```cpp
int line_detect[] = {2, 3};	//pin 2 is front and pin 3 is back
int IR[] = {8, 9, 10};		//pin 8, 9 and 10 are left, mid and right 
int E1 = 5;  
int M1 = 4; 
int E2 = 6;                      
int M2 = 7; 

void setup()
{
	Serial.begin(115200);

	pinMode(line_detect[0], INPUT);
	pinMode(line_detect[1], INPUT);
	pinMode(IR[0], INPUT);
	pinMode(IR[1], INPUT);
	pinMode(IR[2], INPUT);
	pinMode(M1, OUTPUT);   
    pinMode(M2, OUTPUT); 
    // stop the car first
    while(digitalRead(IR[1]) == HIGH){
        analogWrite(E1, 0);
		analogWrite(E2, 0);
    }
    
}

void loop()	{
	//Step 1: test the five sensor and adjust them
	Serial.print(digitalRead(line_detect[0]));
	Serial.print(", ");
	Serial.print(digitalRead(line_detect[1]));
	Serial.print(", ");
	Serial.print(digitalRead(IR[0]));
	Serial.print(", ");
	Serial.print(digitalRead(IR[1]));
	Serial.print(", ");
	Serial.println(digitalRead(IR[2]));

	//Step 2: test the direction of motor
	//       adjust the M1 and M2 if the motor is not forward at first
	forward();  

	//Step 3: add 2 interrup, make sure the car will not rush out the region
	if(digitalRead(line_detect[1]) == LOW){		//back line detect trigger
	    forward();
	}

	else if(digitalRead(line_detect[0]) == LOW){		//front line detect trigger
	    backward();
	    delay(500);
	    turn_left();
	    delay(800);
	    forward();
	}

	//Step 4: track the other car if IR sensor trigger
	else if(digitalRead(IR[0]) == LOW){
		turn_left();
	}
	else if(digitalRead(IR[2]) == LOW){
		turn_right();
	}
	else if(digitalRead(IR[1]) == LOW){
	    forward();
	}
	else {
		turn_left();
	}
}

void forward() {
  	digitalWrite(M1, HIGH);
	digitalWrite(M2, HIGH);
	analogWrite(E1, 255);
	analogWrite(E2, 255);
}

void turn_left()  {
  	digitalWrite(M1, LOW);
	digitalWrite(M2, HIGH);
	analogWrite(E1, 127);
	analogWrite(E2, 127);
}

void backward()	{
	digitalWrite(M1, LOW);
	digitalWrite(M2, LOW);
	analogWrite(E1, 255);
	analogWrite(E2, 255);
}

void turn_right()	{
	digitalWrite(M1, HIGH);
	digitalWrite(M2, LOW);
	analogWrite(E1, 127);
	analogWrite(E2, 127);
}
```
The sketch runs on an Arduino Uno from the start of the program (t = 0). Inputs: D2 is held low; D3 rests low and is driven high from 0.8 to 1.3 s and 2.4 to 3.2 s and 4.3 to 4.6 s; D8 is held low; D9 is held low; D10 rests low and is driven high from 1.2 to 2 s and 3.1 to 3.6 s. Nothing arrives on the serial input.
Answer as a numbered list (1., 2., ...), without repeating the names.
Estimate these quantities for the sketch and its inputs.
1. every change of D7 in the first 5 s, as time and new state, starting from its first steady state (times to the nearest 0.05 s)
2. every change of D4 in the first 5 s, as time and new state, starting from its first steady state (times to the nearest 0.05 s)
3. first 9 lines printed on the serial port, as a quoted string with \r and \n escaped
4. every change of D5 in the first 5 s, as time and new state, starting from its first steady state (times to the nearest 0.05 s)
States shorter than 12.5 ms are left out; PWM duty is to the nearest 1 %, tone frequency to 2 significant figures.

1. 0 s high; 0.8 s low; 1.3 s high; 2.4 s low; 2.9 s high; 4.3 s low; 4.8 s high
2. 0 s high; 0.8 s low; 2.1 s high; 2.4 s low; 3.7 s high; 4.3 s low
3. "0, 0, 0, 0, 0\r\n0, 0, 0, 0, 0\r\n0, 0, 0, 0, 0\r\n0, 0, 0, 0, 0\r\n0, 0, 0, 0, 0\r\n0, 0, 0, 0, 0\r\n0, 0, 0, 0, 0\r\n0, 0, 0, 0, 0\r\n0, 0, 0, 0, 0\r\n"
4. 0 s high; 1.3 s PWM 50 %; 2.1 s high; 2.9 s PWM 50 %; 3.7 s high; 4.8 s PWM 50 %
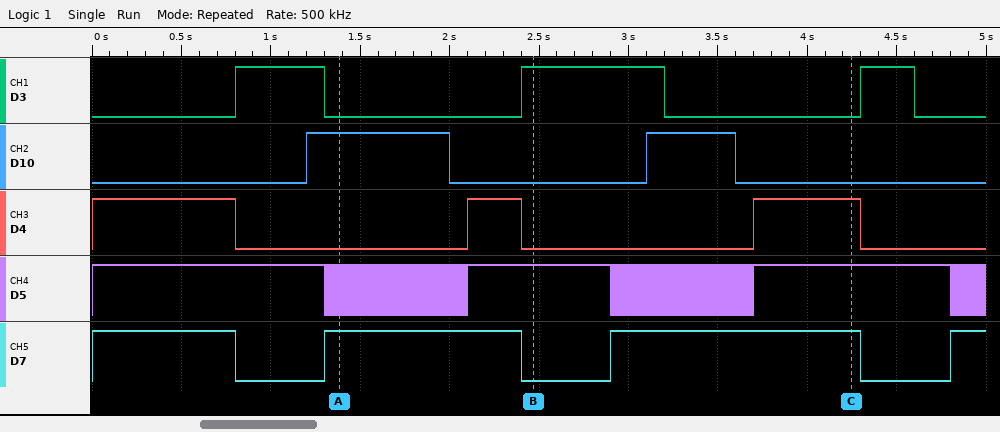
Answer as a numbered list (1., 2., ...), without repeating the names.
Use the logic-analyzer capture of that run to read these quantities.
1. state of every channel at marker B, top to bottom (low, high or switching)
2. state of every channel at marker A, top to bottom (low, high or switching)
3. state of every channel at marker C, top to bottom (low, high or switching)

1. D3 high, D10 low, D4 low, D5 high, D7 low
2. D3 low, D10 high, D4 low, D5 switching, D7 high
3. D3 low, D10 low, D4 high, D5 high, D7 high
